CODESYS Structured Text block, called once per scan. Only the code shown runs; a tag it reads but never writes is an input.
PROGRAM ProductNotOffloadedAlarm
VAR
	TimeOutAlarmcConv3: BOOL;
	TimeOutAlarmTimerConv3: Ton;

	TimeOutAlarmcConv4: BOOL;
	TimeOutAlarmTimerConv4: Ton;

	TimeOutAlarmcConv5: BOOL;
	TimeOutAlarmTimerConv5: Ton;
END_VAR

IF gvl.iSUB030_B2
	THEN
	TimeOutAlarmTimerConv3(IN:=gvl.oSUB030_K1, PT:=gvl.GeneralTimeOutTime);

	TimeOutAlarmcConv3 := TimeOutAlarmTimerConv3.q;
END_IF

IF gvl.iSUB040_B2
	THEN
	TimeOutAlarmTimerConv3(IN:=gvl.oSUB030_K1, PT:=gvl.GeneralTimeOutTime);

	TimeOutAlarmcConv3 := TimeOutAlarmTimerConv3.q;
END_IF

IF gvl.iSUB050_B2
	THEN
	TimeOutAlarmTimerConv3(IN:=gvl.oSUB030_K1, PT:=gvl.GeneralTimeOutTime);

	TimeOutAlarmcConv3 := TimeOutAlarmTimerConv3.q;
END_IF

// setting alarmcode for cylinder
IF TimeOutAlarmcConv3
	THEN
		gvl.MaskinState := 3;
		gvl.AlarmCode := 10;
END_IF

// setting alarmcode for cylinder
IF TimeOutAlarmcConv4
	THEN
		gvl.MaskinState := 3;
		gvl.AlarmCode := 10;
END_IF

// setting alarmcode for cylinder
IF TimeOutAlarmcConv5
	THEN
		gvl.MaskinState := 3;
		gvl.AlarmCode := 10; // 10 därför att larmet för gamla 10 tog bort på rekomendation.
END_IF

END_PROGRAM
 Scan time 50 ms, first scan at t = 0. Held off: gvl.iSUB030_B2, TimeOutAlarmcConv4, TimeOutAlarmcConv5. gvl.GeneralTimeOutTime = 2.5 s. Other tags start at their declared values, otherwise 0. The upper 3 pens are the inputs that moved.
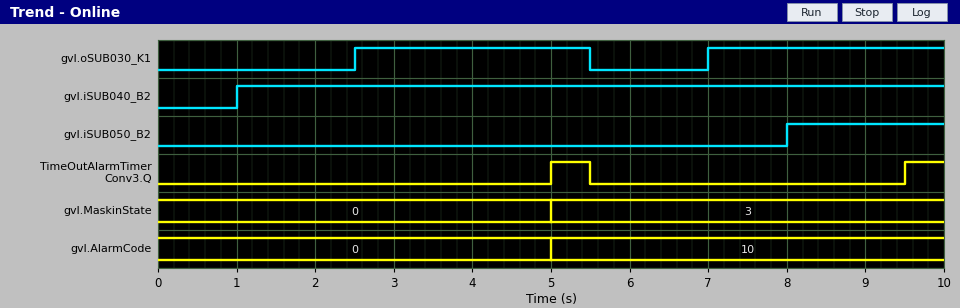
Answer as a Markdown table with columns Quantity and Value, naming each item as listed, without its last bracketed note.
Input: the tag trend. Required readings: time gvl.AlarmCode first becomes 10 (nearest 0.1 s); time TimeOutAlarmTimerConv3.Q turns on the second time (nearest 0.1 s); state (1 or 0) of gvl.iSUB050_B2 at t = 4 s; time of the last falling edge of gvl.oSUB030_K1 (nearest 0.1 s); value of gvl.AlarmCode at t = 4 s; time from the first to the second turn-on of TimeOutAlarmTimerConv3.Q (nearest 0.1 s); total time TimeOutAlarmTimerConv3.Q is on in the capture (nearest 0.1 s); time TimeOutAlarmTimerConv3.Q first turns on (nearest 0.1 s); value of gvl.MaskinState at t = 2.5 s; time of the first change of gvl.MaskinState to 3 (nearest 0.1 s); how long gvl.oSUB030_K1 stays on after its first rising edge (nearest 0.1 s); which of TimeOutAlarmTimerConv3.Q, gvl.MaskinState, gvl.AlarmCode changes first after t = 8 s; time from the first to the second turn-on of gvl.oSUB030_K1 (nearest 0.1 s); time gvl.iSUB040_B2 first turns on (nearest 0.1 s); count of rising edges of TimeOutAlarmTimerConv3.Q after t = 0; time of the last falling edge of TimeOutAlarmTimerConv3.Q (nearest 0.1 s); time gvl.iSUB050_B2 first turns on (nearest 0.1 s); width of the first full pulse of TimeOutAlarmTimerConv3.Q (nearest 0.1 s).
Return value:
| Quantity | Value |
|---|---|
| time gvl.AlarmCode first becomes 10 | 5.0 s |
| time TimeOutAlarmTimerConv3.Q turns on the second time | 9.5 s |
| state (1 or 0) of gvl.iSUB050_B2 at t = 4 s | 0 |
| time of the last falling edge of gvl.oSUB030_K1 | 5.5 s |
| value of gvl.AlarmCode at t = 4 s | 0 |
| time from the first to the second turn-on of TimeOutAlarmTimerConv3.Q | 4.5 s |
| total time TimeOutAlarmTimerConv3.Q is on in the capture | 1.0 s |
| time TimeOutAlarmTimerConv3.Q first turns on | 5.0 s |
| value of gvl.MaskinState at t = 2.5 s | 0 |
| time of the first change of gvl.MaskinState to 3 | 5.0 s |
| how long gvl.oSUB030_K1 stays on after its first rising edge | 3.0 s |
| which of TimeOutAlarmTimerConv3.Q, gvl.MaskinState, gvl.AlarmCode changes first after t = 8 s | TimeOutAlarmTimerConv3.Q |
| time from the first to the second turn-on of gvl.oSUB030_K1 | 4.5 s |
| time gvl.iSUB040_B2 first turns on | 1.0 s |
| count of rising edges of TimeOutAlarmTimerConv3.Q after t = 0 | 2 |
| time of the last falling edge of TimeOutAlarmTimerConv3.Q | 5.5 s |
| time gvl.iSUB050_B2 first turns on | 8.0 s |
| width of the first full pulse of TimeOutAlarmTimerConv3.Q | 0.5 s |
